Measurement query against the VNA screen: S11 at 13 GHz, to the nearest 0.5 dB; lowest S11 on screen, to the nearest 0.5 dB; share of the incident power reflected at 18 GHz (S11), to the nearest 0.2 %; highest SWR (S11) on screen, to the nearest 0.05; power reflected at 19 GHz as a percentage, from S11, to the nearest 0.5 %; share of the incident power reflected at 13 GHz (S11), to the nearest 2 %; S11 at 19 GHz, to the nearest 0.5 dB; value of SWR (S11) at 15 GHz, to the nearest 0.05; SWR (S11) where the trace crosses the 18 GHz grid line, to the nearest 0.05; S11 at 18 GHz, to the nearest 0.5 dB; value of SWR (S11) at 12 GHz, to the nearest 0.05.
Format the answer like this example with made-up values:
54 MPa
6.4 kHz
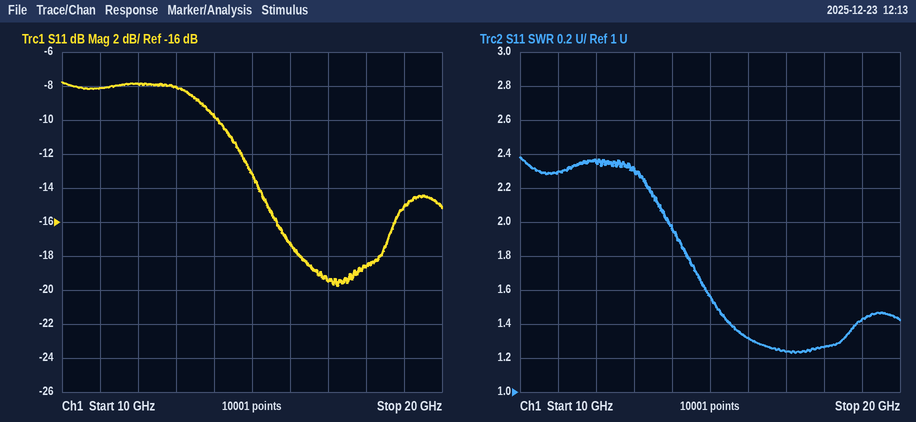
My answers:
-8.0 dB
-20.0 dB
1.4 %
2.40
3.0 %
16 %
-15.0 dB
1.55
1.25
-18.5 dB
2.35
